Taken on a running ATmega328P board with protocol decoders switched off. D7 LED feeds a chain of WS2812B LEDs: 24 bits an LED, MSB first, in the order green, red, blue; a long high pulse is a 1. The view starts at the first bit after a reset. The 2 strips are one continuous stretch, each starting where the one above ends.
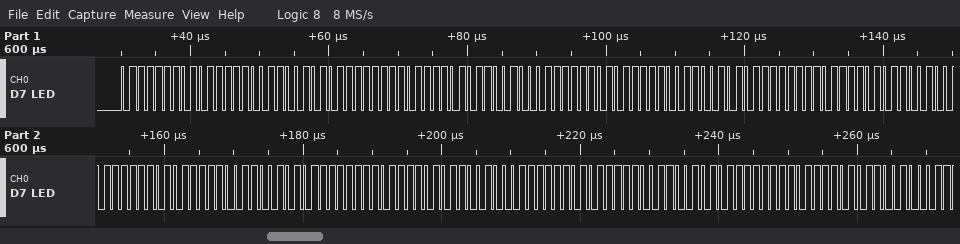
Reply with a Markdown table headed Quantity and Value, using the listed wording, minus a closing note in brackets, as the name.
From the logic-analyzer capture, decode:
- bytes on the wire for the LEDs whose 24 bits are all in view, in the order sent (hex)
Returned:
| Quantity | Value |
|---|---|
| bytes on the wire for the LEDs whose 24 bits are all in view, in the order sent | 7E BE 65 7F BD 64 7E BE 65 7F BD 64 7E BE 65 7F BD 64 7E BE 65 7F BD 64 |
